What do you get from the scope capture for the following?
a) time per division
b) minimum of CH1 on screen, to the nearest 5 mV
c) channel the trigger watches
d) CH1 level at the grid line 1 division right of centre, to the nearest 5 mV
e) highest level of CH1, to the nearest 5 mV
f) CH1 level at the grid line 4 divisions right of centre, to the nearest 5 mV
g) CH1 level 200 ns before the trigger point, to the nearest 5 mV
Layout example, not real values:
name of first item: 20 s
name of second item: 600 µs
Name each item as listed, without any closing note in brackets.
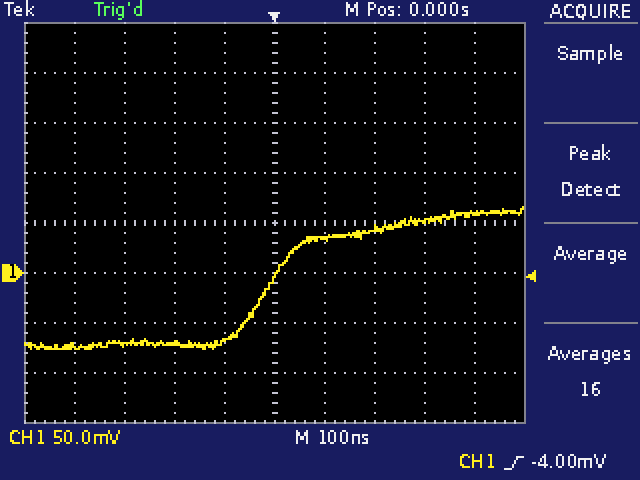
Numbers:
time per division: 100 ns
minimum of CH1 on screen, to the nearest 5 mV: -75 mV
channel the trigger watches: CH1
CH1 level at the grid line 1 division right of centre, to the nearest 5 mV: 35 mV
highest level of CH1, to the nearest 5 mV: 65 mV
CH1 level at the grid line 4 divisions right of centre, to the nearest 5 mV: 60 mV
CH1 level 200 ns before the trigger point, to the nearest 5 mV: -70 mV
